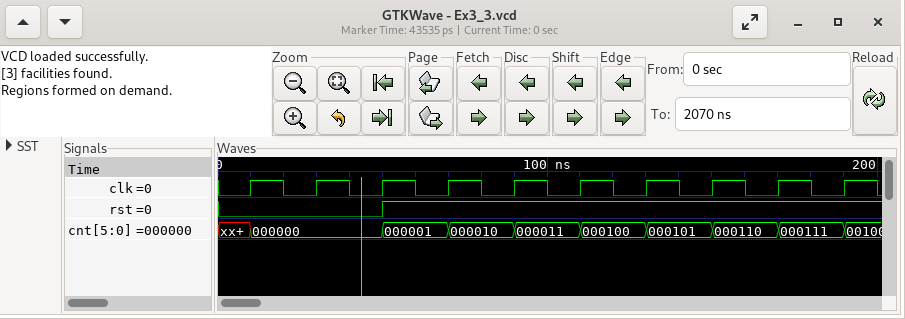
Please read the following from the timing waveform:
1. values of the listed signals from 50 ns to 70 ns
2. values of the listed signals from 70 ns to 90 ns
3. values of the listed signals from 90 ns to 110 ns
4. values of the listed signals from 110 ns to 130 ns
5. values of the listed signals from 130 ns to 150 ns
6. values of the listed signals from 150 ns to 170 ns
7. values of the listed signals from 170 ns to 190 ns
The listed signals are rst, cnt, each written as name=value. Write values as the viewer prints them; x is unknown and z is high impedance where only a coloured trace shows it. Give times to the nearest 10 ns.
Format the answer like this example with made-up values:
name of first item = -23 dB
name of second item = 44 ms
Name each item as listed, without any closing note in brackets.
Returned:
values of the listed signals from 50 ns to 70 ns = rst=1, cnt=000001
values of the listed signals from 70 ns to 90 ns = rst=1, cnt=000010
values of the listed signals from 90 ns to 110 ns = rst=1, cnt=000011
values of the listed signals from 110 ns to 130 ns = rst=1, cnt=000100
values of the listed signals from 130 ns to 150 ns = rst=1, cnt=000101
values of the listed signals from 150 ns to 170 ns = rst=1, cnt=000110
values of the listed signals from 170 ns to 190 ns = rst=1, cnt=000111
